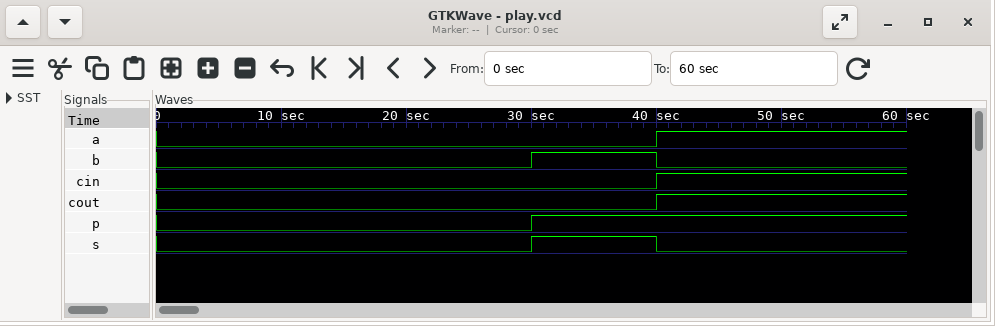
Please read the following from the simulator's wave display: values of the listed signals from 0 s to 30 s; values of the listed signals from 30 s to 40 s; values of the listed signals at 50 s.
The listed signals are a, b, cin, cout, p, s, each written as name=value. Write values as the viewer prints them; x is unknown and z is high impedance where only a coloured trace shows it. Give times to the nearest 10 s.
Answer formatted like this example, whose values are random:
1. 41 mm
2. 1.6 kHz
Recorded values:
1. a=0, b=0, cin=0, cout=0, p=0, s=0
2. a=0, b=1, cin=0, cout=0, p=1, s=1
3. a=1, b=0, cin=1, cout=1, p=1, s=0
